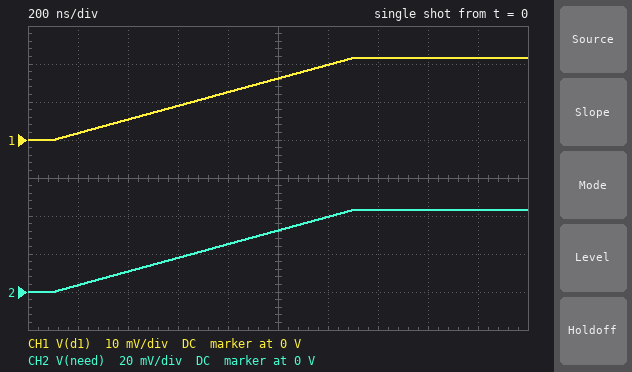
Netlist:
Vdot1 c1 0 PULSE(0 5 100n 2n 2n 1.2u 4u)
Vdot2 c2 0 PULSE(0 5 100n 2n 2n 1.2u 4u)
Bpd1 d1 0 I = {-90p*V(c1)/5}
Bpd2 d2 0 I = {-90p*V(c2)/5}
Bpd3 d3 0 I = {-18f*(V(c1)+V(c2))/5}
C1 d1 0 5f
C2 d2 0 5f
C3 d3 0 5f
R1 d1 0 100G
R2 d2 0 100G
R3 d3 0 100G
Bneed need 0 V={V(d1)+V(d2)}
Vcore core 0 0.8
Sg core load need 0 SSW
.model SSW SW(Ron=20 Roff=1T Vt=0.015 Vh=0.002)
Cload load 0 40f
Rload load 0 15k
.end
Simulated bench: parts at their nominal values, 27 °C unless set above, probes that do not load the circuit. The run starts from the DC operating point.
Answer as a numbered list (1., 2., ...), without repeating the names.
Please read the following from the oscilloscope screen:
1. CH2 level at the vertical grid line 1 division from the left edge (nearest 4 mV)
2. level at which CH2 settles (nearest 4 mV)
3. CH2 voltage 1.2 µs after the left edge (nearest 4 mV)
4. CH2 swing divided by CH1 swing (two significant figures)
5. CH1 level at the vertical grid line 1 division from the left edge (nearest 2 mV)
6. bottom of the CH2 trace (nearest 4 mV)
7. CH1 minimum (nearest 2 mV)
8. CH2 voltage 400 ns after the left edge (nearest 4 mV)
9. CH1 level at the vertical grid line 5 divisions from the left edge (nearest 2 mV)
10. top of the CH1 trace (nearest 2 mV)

1. 4 mV
2. 44 mV
3. 40 mV
4. 2.0
5. 2 mV
6. 0 V
7. 0 V
8. 12 mV
9. 16 mV
10. 22 mV
